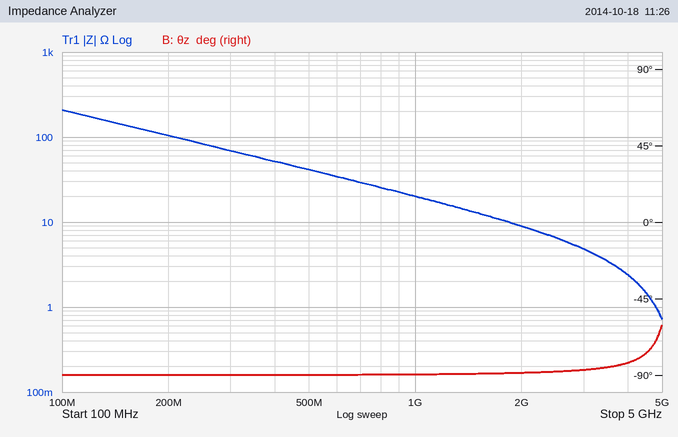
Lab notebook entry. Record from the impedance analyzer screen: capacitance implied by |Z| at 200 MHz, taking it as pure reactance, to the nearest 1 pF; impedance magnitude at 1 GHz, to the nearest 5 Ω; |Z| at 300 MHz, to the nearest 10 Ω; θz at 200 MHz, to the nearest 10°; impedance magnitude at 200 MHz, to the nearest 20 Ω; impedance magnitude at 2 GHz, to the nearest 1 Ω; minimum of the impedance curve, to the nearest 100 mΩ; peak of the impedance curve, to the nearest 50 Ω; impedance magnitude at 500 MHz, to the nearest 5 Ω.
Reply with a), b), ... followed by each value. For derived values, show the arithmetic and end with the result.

a) C = 1/(2π × 200 MHz × 100 Ω) ≈ 8 pF
b) 20 Ω
c) 70 Ω
d) -90°
e) 100 Ω
f) 9 Ω
g) 700 mΩ
h) 200 Ω
i) 40 Ω
